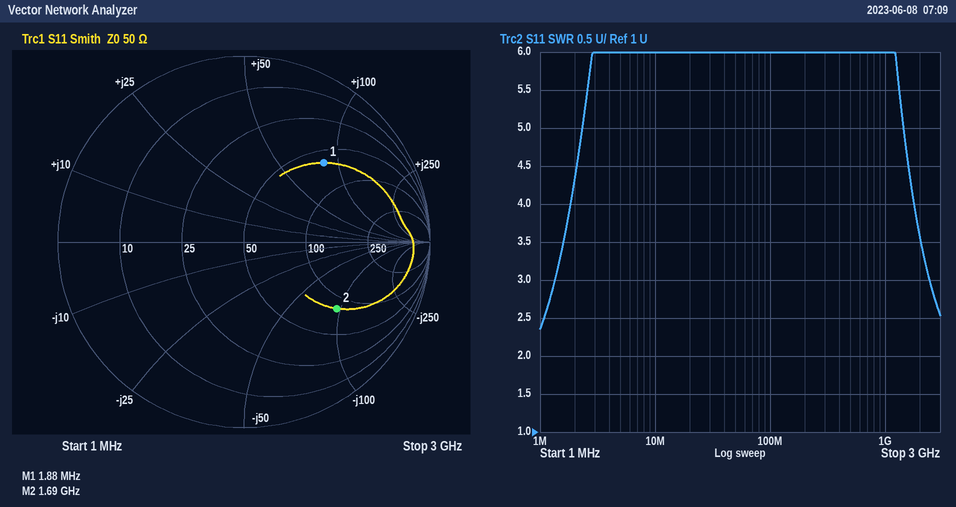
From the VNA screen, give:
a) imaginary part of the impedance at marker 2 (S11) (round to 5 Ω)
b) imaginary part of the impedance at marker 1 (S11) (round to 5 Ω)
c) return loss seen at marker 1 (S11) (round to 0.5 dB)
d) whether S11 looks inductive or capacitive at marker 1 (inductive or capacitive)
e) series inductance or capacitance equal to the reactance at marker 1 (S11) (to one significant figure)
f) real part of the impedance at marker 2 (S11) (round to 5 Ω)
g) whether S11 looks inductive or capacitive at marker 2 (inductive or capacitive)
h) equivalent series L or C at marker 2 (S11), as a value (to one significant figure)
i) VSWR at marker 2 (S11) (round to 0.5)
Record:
-95 Ω
+85 Ω
4.5 dB
inductive
7 µH
80 Ω
capacitive
1.0 pF
4.0
